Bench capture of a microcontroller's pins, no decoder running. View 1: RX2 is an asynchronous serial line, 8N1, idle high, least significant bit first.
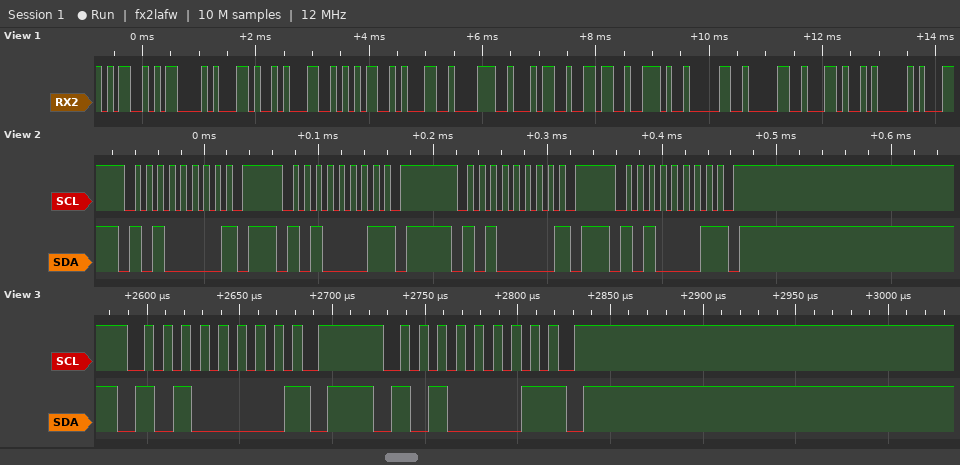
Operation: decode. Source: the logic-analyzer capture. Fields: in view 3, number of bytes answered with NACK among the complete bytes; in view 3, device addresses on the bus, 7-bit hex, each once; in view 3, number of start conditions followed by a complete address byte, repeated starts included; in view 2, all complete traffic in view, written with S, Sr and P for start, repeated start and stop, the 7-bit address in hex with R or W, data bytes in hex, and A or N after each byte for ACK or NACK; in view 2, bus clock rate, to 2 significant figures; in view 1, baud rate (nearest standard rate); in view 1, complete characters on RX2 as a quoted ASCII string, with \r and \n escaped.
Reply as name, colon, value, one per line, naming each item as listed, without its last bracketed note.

in view 3, number of bytes answered with NACK among the complete bytes: 2
in view 3, device addresses on the bus, 7-bit hex, each once: 0x50
in view 3, number of start conditions followed by a complete address byte, repeated starts included: 2
in view 2, all complete traffic in view, written with S, Sr and P for start, repeated start and stop, the 7-bit address in hex with R or W, data bytes in hex, and A or N after each byte for ACK or NACK: S 50W N P S 50R N P S 50W N P S 50R N P
in view 2, bus clock rate, to 2 significant figures: 100 kHz
in view 1, baud rate: 9600 baud
in view 1, complete characters on RX2 as a quoted ASCII string, with \r and \n escaped: "MC,151846.00,A"
